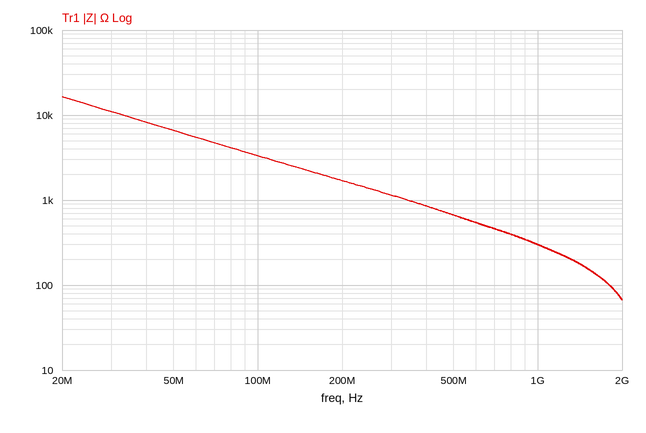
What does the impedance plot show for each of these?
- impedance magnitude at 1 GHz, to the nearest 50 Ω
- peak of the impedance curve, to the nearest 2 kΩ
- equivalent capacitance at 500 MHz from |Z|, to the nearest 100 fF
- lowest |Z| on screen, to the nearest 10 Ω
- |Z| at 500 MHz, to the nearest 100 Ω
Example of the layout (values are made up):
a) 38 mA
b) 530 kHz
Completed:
a) 300 Ω
b) 16 kΩ
c) 500 fF
d) 70 Ω
e) 700 Ω
